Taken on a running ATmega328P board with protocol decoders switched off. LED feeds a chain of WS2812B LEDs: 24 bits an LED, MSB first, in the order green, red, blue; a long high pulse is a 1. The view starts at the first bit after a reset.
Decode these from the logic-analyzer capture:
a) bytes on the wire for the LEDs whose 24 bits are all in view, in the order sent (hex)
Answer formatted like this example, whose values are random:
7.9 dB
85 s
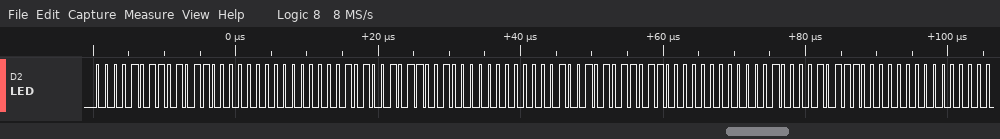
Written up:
0B 58 00 0A 59 00 09 5B 00 08 5C 00
